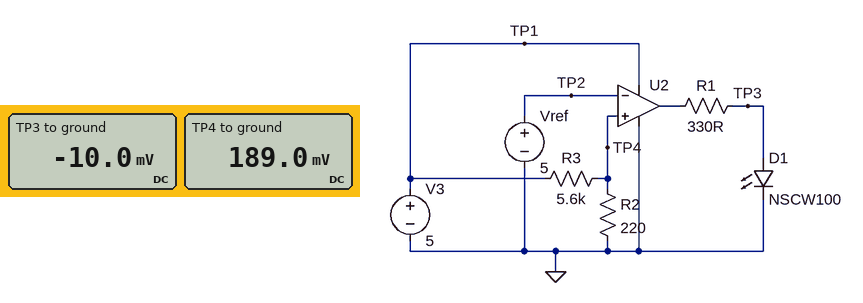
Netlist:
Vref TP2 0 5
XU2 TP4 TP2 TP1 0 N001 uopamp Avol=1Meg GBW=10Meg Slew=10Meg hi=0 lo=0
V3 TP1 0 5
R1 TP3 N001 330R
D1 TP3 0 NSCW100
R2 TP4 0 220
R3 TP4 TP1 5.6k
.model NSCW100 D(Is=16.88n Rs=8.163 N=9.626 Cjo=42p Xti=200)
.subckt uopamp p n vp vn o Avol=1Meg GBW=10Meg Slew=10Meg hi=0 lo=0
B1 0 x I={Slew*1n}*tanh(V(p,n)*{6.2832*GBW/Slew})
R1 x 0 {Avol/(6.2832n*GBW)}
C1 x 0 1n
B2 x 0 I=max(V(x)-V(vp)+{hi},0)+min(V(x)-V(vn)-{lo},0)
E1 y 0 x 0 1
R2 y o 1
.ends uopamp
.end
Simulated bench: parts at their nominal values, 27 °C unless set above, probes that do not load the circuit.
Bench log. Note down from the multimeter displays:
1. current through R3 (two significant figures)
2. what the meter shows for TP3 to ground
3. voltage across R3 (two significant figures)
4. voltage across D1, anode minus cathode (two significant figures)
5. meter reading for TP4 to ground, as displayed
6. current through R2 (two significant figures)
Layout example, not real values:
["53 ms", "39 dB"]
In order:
["860 µA", "-10.0 mV", "4.8 V", "-10 mV", "189.0 mV", "860 µA"]
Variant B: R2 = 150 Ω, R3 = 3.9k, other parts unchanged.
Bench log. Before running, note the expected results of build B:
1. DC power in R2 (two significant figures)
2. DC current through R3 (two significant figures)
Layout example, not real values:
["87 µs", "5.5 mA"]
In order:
["230 µW", "1.2 mA"]
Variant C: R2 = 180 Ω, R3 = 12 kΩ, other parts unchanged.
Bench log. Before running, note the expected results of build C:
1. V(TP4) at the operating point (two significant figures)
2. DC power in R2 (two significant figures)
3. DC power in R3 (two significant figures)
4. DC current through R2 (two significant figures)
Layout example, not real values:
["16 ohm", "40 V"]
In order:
["74 mV", "30 µW", "2.0 mW", "410 µA"]
